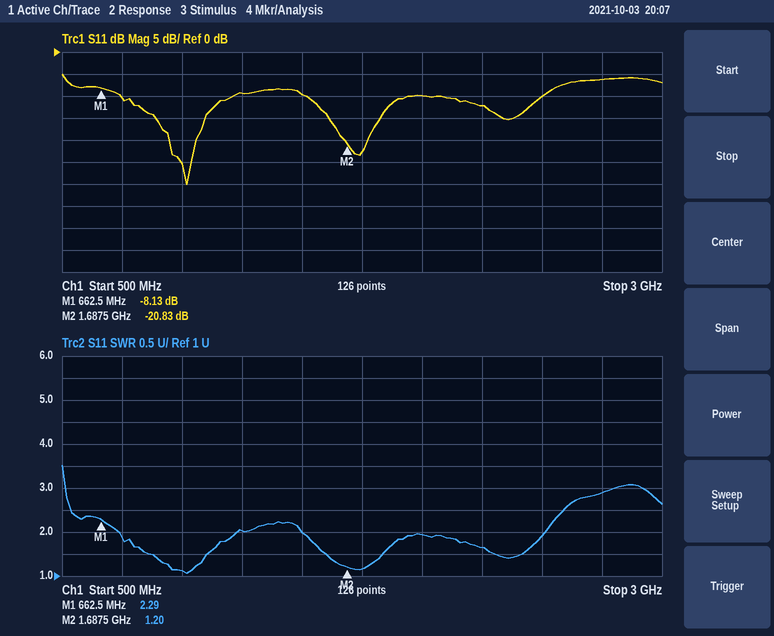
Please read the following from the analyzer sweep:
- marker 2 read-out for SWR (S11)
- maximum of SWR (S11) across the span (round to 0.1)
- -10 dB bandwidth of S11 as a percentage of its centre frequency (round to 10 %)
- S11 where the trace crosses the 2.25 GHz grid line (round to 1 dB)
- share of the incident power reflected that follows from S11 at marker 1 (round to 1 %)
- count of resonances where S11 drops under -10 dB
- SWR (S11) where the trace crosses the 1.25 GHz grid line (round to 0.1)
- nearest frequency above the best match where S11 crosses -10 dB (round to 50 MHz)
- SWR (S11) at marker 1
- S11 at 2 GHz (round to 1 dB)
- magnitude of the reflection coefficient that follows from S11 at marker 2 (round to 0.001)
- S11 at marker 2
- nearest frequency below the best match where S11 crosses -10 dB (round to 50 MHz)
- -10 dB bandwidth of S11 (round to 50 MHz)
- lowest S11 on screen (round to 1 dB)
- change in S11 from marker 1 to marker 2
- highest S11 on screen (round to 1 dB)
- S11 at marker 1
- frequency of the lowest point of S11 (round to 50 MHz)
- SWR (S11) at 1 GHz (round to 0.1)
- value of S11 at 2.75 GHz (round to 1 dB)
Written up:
1.20
3.5
50 %
-12 dB
15 %
3
2.0
1.20 GHz
2.29
-10 dB
0.091
-20.83 dB
750 MHz
450 MHz
-30 dB
-12.70 dB
-5 dB
-8.13 dB
1.00 GHz
1.1
-6 dB
